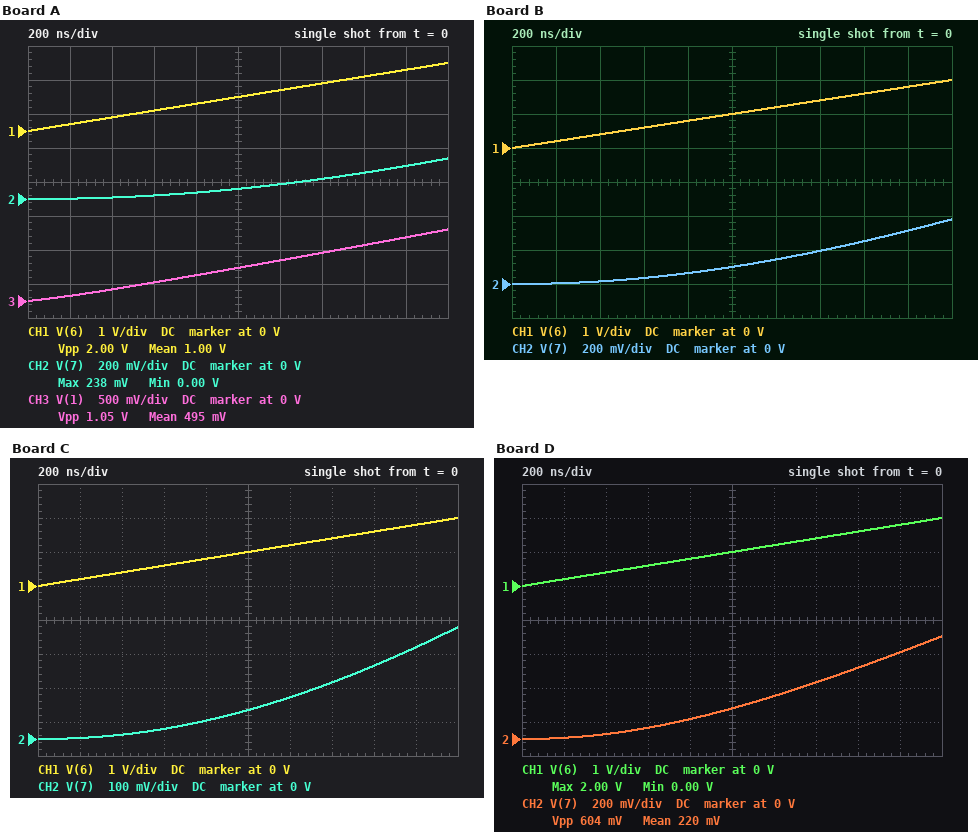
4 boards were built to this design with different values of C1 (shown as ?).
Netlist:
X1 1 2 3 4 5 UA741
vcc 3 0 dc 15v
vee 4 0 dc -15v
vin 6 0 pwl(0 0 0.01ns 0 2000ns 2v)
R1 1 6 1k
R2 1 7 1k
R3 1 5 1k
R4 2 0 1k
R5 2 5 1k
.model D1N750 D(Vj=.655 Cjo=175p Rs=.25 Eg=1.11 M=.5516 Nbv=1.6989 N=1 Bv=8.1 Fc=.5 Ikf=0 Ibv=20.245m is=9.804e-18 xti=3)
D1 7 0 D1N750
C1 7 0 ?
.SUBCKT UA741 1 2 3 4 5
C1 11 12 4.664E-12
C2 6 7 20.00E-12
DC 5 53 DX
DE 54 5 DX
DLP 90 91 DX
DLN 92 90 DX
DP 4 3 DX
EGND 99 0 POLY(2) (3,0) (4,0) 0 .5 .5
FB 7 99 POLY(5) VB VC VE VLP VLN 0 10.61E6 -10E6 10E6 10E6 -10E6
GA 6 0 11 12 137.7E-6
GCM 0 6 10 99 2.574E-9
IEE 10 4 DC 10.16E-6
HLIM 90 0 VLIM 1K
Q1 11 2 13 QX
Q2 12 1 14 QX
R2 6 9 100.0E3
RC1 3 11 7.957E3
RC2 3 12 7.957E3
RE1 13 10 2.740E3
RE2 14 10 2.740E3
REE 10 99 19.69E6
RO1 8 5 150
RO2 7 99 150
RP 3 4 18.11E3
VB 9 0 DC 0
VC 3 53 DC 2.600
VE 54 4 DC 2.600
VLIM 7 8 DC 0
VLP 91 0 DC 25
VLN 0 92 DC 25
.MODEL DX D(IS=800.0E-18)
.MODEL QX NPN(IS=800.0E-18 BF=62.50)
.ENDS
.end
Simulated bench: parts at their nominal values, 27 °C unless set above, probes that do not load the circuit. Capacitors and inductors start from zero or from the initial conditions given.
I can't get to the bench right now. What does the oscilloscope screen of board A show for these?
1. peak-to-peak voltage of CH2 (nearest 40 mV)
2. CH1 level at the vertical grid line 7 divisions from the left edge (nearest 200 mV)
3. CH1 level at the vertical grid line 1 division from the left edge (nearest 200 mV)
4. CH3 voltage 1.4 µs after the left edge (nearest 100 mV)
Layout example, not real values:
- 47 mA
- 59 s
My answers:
- 240 mV
- 1.4 V
- 200 mV
- 700 mV
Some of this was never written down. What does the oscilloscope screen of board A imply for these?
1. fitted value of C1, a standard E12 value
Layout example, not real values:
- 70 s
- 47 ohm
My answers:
- 3.3 nF
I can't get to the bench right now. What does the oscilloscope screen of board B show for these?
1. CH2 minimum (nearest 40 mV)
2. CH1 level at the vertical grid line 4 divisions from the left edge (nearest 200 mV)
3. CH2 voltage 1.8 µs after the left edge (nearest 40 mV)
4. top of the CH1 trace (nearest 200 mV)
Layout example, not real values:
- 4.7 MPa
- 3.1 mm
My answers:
- 0 V
- 800 mV
- 320 mV
- 2.0 V
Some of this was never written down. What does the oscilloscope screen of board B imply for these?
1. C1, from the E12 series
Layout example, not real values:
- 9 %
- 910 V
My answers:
- 1.8 nF
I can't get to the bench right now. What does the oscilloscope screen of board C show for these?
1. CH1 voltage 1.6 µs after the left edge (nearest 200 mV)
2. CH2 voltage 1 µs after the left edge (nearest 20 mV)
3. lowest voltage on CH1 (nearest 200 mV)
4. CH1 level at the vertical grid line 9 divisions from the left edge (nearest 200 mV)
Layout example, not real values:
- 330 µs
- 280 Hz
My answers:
- 1.6 V
- 80 mV
- 0 V
- 1.8 V
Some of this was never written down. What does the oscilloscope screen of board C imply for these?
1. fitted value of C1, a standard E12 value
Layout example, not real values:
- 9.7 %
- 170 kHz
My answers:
- 2.2 nF
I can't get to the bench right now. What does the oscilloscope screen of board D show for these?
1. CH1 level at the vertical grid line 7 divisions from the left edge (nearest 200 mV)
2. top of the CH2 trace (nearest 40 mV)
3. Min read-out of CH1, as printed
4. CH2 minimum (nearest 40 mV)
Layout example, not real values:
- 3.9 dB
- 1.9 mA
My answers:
- 1.4 V
- 600 mV
- 0.00 V
- 0 V
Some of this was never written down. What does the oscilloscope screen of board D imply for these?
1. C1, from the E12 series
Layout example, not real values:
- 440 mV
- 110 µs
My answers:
- 820 pF
